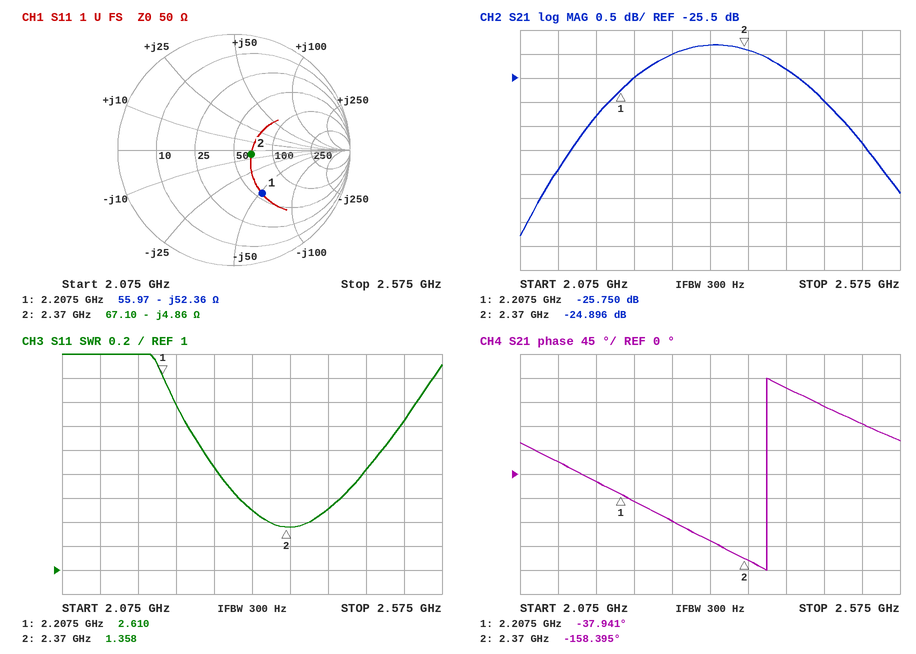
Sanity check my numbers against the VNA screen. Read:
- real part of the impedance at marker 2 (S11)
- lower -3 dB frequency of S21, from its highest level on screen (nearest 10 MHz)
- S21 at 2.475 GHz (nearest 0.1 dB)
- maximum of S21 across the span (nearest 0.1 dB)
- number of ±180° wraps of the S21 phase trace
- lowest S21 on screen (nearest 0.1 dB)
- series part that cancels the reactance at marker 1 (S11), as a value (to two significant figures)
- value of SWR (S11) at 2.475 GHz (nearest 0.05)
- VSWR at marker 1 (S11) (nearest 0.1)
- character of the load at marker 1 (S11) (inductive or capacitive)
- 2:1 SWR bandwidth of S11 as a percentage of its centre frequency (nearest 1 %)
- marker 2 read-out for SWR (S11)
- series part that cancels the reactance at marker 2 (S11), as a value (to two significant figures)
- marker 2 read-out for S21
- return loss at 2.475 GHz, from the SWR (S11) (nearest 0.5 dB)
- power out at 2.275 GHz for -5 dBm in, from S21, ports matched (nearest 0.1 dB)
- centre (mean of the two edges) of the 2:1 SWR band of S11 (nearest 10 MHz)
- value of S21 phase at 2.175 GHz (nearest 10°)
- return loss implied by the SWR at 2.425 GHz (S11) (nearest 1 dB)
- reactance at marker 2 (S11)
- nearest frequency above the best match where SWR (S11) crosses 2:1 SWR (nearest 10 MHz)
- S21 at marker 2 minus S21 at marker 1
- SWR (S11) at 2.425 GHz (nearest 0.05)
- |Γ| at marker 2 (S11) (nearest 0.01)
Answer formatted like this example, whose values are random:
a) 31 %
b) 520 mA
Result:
a) 67.10 Ω
b) 2.11 GHz
c) -26.0 dB
d) -24.8 dB
e) 1
f) -28.8 dB
g) 3.8 nH
h) 1.85
i) 2.6
j) capacitive
k) 10 %
l) 1.358
m) 330 pH
n) -24.896 dB
o) 10.5 dB
p) -30.0 dBm
q) 2.38 GHz
r) -10°
s) 14 dB
t) -4.86 Ω
u) 2.50 GHz
v) 0.854 dB
w) 1.50
x) 0.15
